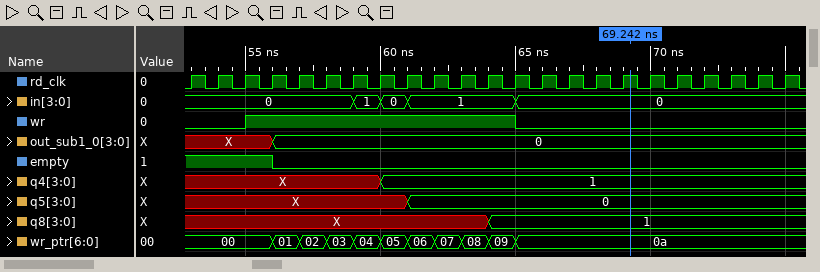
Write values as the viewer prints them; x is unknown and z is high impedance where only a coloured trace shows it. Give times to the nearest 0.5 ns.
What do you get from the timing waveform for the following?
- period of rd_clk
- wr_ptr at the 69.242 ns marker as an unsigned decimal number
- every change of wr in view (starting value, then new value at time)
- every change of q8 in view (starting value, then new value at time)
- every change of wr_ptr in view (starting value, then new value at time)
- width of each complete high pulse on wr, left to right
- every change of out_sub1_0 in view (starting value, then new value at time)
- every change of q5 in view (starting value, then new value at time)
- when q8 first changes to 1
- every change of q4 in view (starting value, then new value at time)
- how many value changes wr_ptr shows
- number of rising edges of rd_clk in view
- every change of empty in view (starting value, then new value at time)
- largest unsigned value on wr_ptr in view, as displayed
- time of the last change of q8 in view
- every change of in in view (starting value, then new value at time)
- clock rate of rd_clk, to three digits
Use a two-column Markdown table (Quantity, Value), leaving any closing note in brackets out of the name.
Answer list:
| Quantity | Value |
|---|---|
| period of rd_clk | 1 ns |
| wr_ptr at the 69.242 ns marker as an unsigned decimal number | 10 |
| every change of wr in view | 0, 1 at 55 ns, 0 at 65 ns |
| every change of q8 in view | X, 1 at 64 ns |
| every change of wr_ptr in view | 00, 01 at 56 ns, 02 at 57 ns, 03 at 58 ns, 04 at 59 ns, 05 at 60 ns, 06 at 61 ns, 07 at 62 ns, 08 at 63 ns, 09 at 64 ns, 0a at 65 ns |
| width of each complete high pulse on wr, left to right | 10 ns |
| every change of out_sub1_0 in view | X, 0 at 56 ns |
| every change of q5 in view | X, 0 at 61 ns |
| when q8 first changes to 1 | 64 ns |
| every change of q4 in view | X, 1 at 60 ns |
| how many value changes wr_ptr shows | 10 |
| number of rising edges of rd_clk in view | 23 |
| every change of empty in view | 1, 0 at 56 ns |
| largest unsigned value on wr_ptr in view, as displayed | 0a |
| time of the last change of q8 in view | 64 ns |
| every change of in in view | 0, 1 at 59 ns, 0 at 60 ns, 1 at 61 ns, 0 at 65 ns |
| clock rate of rd_clk, to three digits | 1.00 GHz |
